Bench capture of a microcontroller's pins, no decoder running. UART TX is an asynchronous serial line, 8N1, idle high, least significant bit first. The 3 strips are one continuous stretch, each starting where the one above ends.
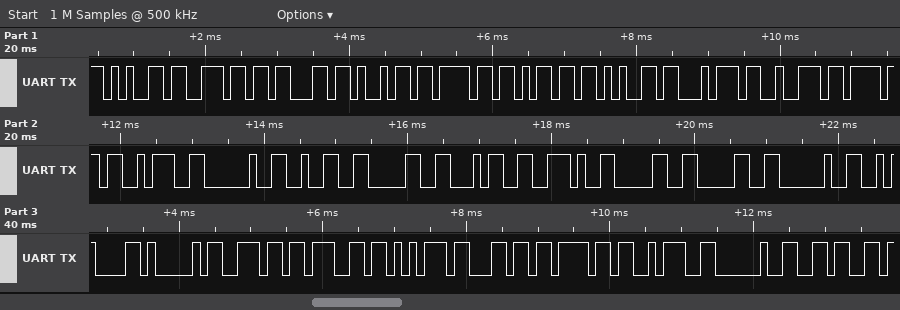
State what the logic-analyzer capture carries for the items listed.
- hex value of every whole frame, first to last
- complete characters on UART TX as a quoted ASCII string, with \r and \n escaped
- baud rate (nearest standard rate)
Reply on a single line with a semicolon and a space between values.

65 6E 63 69 6F 6D 65 74 72 6F 3A 20 32 30 34 2E 30 30 20 0A 41 6E 67 75 6C 6F 3A 20 36; "enciometro: 204.00 \nAngulo: 6"; 9600 baud
